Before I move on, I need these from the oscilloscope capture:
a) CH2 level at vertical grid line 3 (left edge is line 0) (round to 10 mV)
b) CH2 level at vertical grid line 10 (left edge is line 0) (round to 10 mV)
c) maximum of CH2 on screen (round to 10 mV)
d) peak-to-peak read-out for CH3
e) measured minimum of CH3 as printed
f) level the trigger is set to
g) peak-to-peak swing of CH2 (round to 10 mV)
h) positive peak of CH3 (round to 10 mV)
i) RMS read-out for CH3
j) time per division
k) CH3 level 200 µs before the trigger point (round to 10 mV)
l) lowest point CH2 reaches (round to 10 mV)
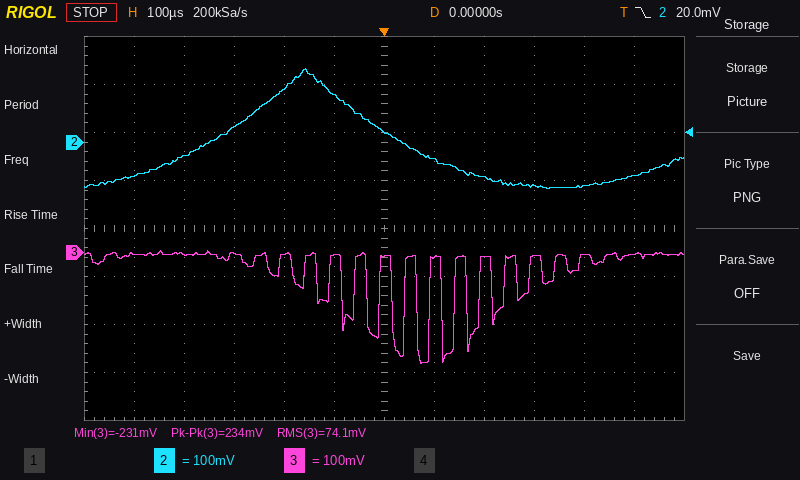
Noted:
30 mV
-90 mV
150 mV
234 mV
-231 mV
20.0 mV
250 mV
0 mV
74.1 mV
100 µs
0 mV
-100 mV
